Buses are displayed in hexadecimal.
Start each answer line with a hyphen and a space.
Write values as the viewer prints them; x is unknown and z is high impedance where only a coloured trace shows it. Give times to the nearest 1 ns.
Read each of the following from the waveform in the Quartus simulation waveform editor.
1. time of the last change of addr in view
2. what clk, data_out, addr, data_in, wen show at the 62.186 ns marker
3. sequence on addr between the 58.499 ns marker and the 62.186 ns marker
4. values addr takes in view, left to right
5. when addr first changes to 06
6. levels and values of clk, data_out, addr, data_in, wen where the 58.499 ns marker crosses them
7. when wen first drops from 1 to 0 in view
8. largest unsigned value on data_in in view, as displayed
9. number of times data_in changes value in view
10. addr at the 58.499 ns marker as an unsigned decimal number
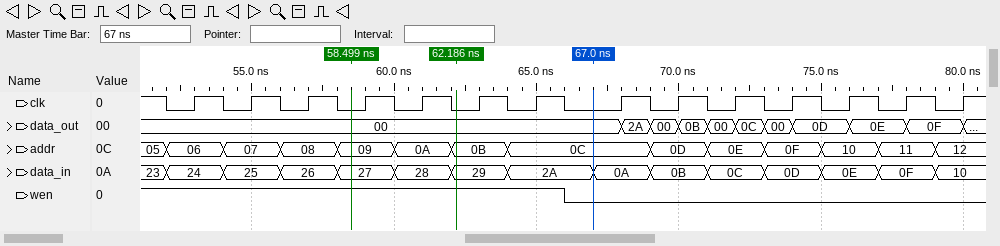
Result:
- 79 ns
- clk=0, data_out=00, addr=0B, data_in=29, wen=1
- 09, 0A, 0B
- 05, 06, 07, 08, 09, 0A, 0B, 0C, 0D, 0E, 0F, 10, 11, 12
- 52 ns
- clk=0, data_out=00, addr=09, data_in=27, wen=1
- 66 ns
- 2A
- 14
- 9
